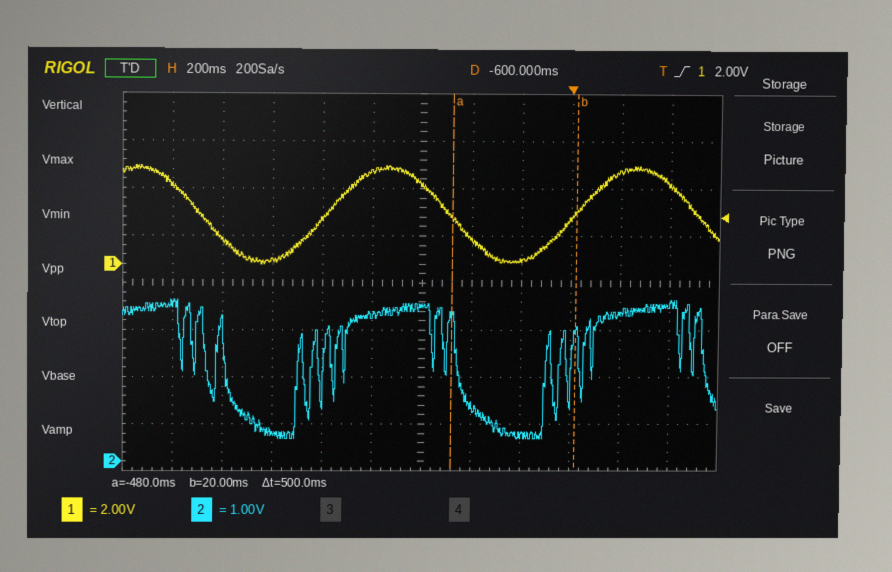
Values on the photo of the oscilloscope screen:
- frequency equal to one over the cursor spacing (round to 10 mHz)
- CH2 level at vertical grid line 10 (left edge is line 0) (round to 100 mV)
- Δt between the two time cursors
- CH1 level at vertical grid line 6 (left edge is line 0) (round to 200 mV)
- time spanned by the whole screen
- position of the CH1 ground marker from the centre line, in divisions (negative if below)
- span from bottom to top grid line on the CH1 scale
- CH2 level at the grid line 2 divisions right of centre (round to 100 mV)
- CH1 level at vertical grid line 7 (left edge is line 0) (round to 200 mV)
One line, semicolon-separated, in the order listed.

2.00 Hz; 3.1 V; 500 ms; 3.4 V; 2.4 s; +0.4 div; 16 V; 600 mV; 1.0 V
